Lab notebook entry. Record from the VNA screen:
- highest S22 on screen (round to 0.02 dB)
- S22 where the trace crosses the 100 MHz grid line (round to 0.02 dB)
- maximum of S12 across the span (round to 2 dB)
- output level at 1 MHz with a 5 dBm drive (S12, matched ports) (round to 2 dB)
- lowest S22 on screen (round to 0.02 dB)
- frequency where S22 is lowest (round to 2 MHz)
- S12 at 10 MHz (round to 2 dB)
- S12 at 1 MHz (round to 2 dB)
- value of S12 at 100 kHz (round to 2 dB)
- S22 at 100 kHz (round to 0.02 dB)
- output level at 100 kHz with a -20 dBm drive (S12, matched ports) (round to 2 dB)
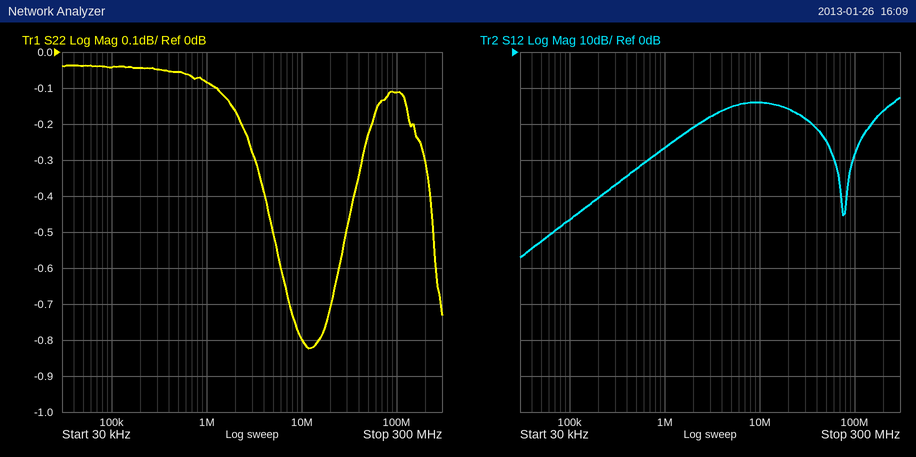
-0.04 dB
-0.12 dB
-12 dB
-22 dBm
-0.82 dB
12 MHz
-14 dB
-26 dB
-46 dB
-0.04 dB
-66 dBm
